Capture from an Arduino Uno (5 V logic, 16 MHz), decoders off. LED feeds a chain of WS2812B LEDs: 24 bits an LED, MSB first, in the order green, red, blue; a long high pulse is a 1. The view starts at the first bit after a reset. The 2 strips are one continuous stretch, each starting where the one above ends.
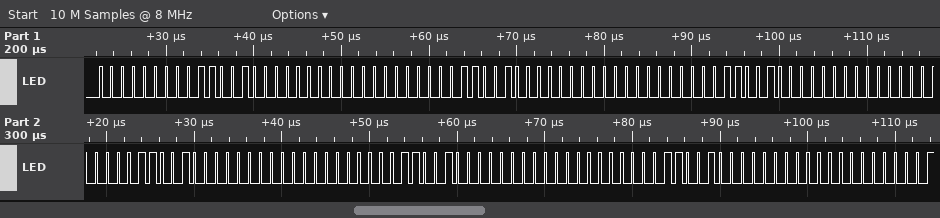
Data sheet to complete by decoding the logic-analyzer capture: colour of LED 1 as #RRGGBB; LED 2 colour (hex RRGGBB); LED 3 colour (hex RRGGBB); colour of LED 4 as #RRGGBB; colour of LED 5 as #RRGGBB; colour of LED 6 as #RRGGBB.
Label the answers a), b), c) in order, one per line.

a) #640000
b) #640000
c) #640000
d) #640000
e) #640000
f) #640000
